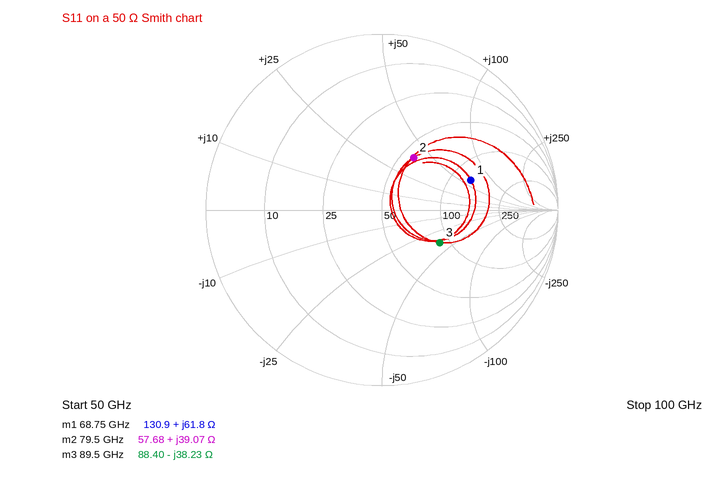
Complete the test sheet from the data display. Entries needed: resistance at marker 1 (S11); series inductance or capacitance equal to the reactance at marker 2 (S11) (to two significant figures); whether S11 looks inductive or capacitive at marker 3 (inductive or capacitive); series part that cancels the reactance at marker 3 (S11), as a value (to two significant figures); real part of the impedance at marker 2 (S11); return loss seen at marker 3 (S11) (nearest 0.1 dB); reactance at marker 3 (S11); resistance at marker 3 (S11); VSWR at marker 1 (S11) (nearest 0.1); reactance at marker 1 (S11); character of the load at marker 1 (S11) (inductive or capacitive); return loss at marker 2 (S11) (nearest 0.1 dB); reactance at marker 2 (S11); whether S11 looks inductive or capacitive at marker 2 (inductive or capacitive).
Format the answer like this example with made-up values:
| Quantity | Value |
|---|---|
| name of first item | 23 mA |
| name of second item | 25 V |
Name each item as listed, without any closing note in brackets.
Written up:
| Quantity | Value |
|---|---|
| resistance at marker 1 | 130.9 Ω |
| series inductance or capacitance equal to the reactance at marker 2 (S11) | 78 pH |
| whether S11 looks inductive or capacitive at marker 3 | capacitive |
| series part that cancels the reactance at marker 3 (S11), as a value | 68 pH |
| real part of the impedance at marker 2 | 57.68 Ω |
| return loss seen at marker 3 (S11) | 8.5 dB |
| reactance at marker 3 | -38.23 Ω |
| resistance at marker 3 | 88.40 Ω |
| VSWR at marker 1 (S11) | 3.3 |
| reactance at marker 1 | +61.8 Ω |
| character of the load at marker 1 (S11) | inductive |
| return loss at marker 2 (S11) | 9.2 dB |
| reactance at marker 2 | +39.07 Ω |
| whether S11 looks inductive or capacitive at marker 2 | inductive |
